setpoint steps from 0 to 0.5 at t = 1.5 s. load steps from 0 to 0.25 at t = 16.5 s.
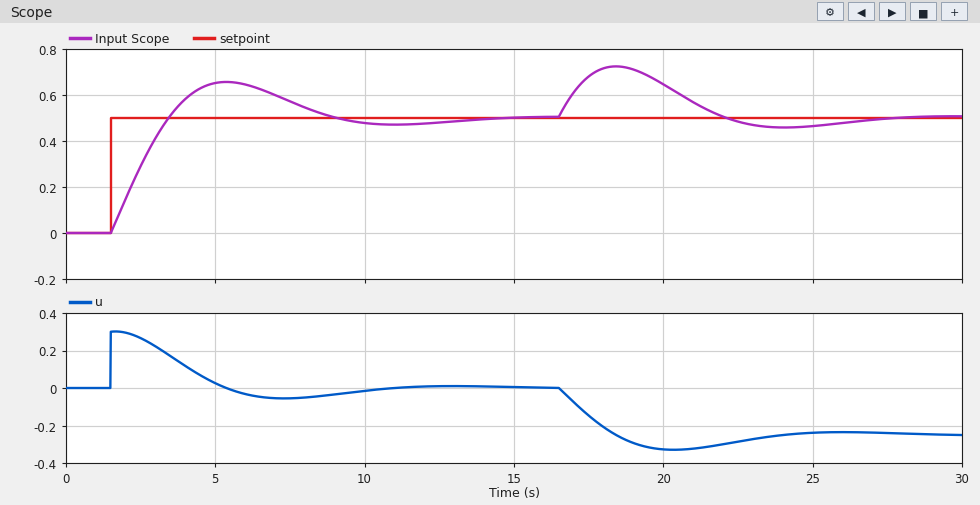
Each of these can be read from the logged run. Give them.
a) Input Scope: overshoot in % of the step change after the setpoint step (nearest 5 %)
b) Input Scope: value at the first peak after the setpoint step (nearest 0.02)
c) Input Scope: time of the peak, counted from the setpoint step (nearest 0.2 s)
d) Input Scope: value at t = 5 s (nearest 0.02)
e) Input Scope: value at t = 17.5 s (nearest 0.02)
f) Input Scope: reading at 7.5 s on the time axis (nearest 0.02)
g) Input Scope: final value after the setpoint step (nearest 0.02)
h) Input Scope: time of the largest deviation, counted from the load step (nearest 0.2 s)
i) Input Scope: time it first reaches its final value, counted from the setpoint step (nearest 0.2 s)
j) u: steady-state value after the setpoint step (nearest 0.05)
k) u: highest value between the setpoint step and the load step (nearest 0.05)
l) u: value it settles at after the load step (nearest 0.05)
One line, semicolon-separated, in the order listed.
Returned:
30 %; 0.66; 3.8 s; 0.66; 0.68; 0.58; 0.50; 2.0 s; 2.0 s; 0.00; 0.30; -0.25
